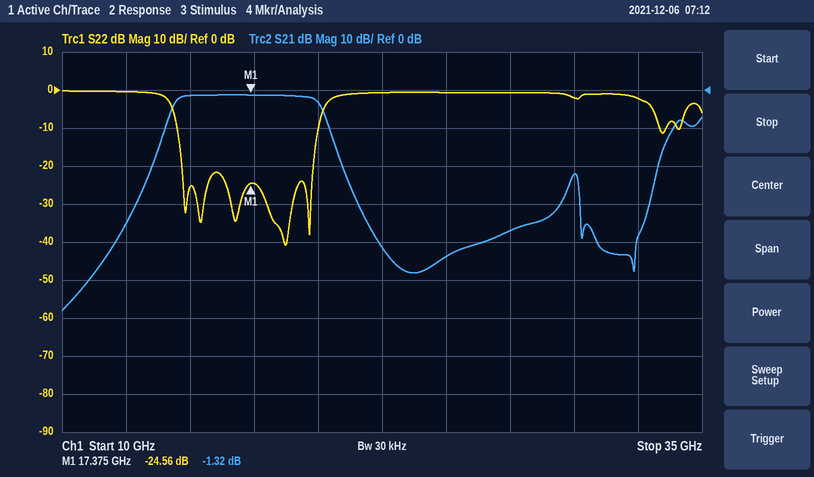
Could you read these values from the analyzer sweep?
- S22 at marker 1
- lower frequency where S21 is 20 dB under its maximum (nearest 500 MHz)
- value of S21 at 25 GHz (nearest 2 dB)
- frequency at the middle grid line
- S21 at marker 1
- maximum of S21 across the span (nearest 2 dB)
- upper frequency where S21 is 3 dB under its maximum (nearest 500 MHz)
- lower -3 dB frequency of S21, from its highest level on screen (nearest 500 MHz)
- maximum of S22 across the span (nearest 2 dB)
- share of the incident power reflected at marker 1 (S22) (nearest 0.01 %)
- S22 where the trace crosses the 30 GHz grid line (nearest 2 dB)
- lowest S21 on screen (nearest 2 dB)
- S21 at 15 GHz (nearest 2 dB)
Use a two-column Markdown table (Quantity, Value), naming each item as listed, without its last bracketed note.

| Quantity | Value |
|---|---|
| S22 at marker 1 | -24.56 dB |
| lower frequency where S21 is 20 dB under its maximum | 13.5 GHz |
| value of S21 at 25 GHz | -44 dB |
| frequency at the middle grid line | 22.5 GHz |
| S21 at marker 1 | -1.32 dB |
| maximum of S21 across the span | -2 dB |
| upper frequency where S21 is 3 dB under its maximum | 20.0 GHz |
| lower -3 dB frequency of S21, from its highest level on screen | 14.5 GHz |
| maximum of S22 across the span | 0 dB |
| share of the incident power reflected at marker 1 (S22) | 0.35 % |
| S22 where the trace crosses the 30 GHz grid line | -2 dB |
| lowest S21 on screen | -58 dB |
| S21 at 15 GHz | -2 dB |
